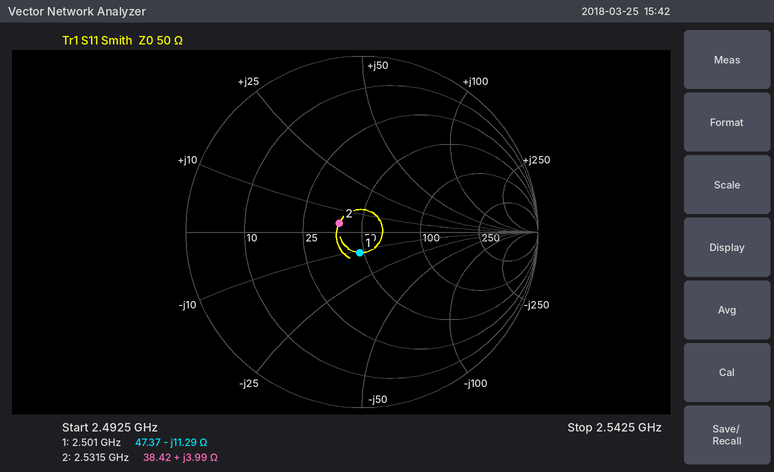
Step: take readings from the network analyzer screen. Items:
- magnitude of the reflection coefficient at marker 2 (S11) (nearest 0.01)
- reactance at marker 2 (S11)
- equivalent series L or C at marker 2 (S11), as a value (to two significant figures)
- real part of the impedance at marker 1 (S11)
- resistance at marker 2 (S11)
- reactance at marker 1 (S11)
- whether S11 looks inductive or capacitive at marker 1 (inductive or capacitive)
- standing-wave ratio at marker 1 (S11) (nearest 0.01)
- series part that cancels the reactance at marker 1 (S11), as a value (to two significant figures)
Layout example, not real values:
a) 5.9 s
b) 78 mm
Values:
a) 0.14
b) +3.99 Ω
c) 250 pH
d) 47.37 Ω
e) 38.42 Ω
f) -11.29 Ω
g) capacitive
h) 1.27
i) 720 pH
